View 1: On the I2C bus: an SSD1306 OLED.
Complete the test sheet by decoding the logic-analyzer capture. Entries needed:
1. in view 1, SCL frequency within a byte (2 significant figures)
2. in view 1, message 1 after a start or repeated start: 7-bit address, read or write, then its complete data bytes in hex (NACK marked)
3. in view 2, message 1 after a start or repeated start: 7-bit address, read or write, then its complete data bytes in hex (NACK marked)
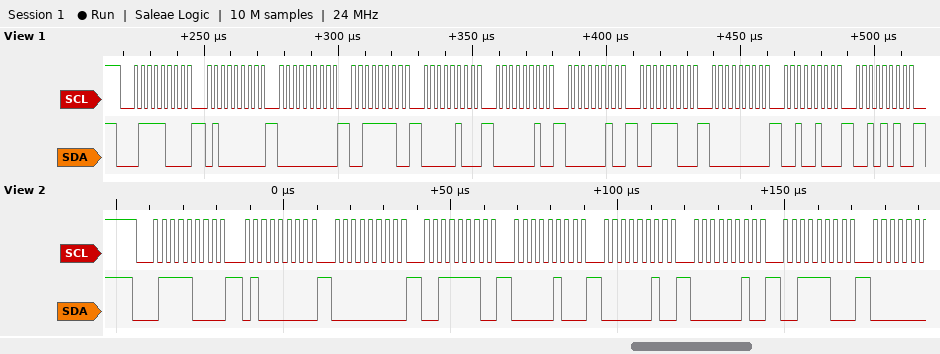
400 kHz
0x3C write: 40 00 3E 04 02 02 3C 00 24 2A
0x3C write: 40 00 3E 04 02 02 3C
